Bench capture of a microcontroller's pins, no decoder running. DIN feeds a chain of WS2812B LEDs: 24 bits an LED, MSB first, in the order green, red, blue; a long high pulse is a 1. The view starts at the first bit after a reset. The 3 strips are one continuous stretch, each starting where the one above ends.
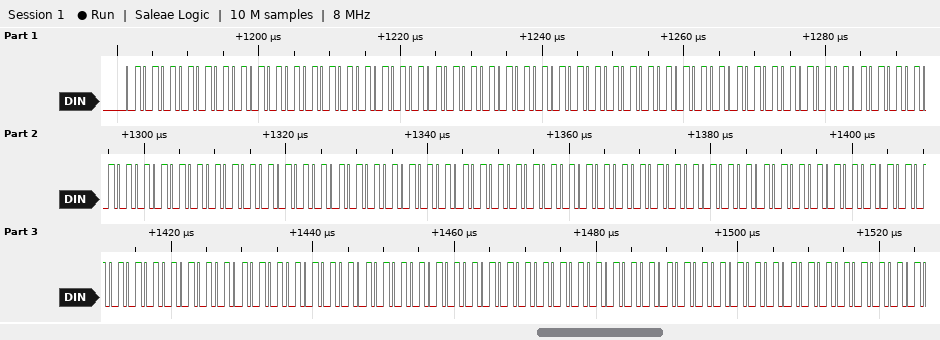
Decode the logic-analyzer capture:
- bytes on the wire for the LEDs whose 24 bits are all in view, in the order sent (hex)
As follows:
55 55 55 55 55 55 55 55 55 55 55 55 55 55 55 55 55 55 55 55 55 55 55 55 55 55 55 55 55 55 55 55 55
